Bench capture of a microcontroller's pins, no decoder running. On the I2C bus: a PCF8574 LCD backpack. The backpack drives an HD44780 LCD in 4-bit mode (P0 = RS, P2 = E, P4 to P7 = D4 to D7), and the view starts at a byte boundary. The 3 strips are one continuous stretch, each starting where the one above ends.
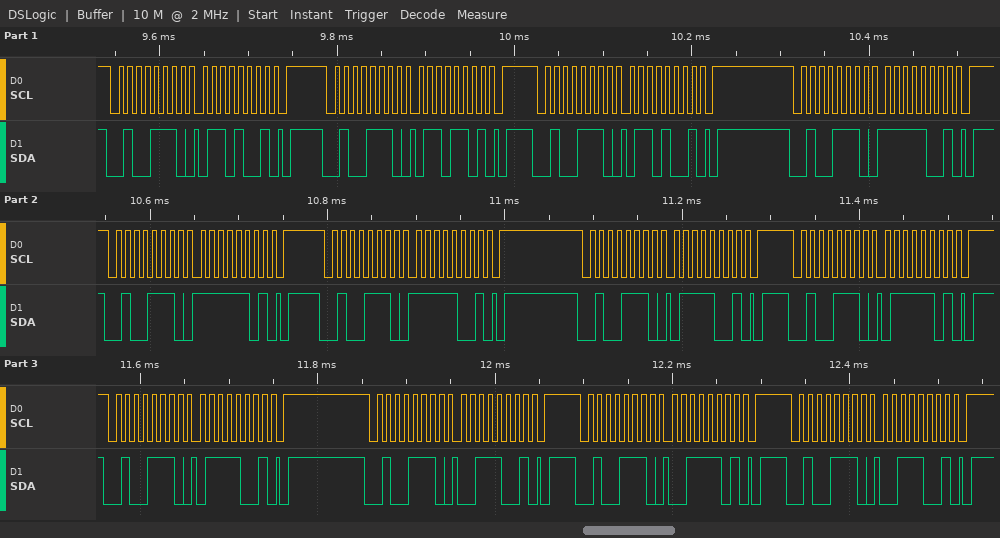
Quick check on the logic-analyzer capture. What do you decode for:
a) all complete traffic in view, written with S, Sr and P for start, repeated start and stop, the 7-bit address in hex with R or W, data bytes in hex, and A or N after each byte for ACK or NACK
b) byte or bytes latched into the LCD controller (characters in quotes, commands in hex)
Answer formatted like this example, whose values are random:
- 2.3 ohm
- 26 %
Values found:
- S 27W A 69 A P S 27W A 6D A P S 27W A 69 A P S 27W A F9 A P S 27W A FD A P S 27W A F9 A P S 27W A 79 A P S 27W A 7D A P S 27W A 79 A P S 27W A 39 A P S 27W A 3D A P S 27W A 39 A P
- 'o' 's'
